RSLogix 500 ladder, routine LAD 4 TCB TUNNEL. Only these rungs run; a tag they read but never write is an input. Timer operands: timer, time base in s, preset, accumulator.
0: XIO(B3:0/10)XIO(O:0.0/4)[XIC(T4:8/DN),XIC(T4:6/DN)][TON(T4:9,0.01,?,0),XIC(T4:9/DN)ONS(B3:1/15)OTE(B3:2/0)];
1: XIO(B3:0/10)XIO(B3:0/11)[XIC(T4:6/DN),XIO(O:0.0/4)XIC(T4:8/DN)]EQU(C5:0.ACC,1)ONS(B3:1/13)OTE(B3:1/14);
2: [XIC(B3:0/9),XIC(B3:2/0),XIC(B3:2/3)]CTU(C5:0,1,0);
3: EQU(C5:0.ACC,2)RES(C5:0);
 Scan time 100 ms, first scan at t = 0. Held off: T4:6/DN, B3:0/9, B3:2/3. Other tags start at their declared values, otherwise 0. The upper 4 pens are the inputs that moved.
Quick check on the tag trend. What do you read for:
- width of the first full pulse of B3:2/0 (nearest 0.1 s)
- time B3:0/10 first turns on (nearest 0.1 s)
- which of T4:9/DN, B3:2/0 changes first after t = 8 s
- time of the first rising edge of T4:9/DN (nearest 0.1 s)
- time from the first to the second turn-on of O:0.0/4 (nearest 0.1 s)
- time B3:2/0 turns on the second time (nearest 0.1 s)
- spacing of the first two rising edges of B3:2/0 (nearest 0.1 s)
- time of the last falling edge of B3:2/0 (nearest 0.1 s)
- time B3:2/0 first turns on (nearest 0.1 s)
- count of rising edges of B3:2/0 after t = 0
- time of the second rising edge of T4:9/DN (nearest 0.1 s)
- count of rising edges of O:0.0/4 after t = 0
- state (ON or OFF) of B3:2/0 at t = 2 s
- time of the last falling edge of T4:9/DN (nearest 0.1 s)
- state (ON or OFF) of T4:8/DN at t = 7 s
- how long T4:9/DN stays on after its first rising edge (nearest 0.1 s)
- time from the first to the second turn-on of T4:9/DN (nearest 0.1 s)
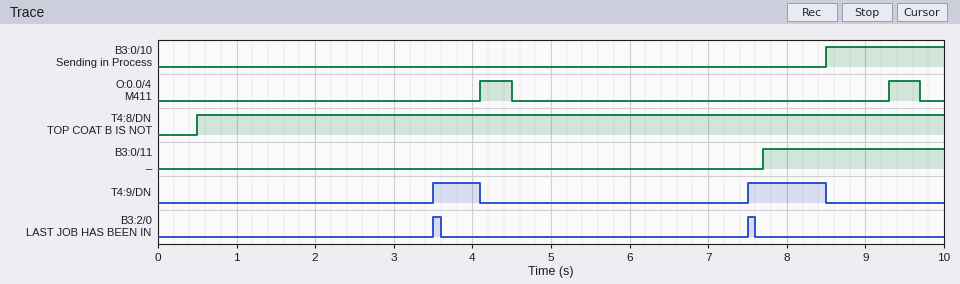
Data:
0.1 s
8.5 s
T4:9/DN
3.5 s
5.2 s
7.5 s
4.0 s
7.6 s
3.5 s
2
7.5 s
2
OFF
8.5 s
ON
0.6 s
4.0 s
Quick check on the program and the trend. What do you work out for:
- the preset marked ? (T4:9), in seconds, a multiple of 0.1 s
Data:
3.0 s
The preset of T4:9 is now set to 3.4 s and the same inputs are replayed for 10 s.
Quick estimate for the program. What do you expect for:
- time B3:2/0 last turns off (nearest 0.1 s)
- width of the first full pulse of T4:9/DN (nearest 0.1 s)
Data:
8.0 s
0.2 s
